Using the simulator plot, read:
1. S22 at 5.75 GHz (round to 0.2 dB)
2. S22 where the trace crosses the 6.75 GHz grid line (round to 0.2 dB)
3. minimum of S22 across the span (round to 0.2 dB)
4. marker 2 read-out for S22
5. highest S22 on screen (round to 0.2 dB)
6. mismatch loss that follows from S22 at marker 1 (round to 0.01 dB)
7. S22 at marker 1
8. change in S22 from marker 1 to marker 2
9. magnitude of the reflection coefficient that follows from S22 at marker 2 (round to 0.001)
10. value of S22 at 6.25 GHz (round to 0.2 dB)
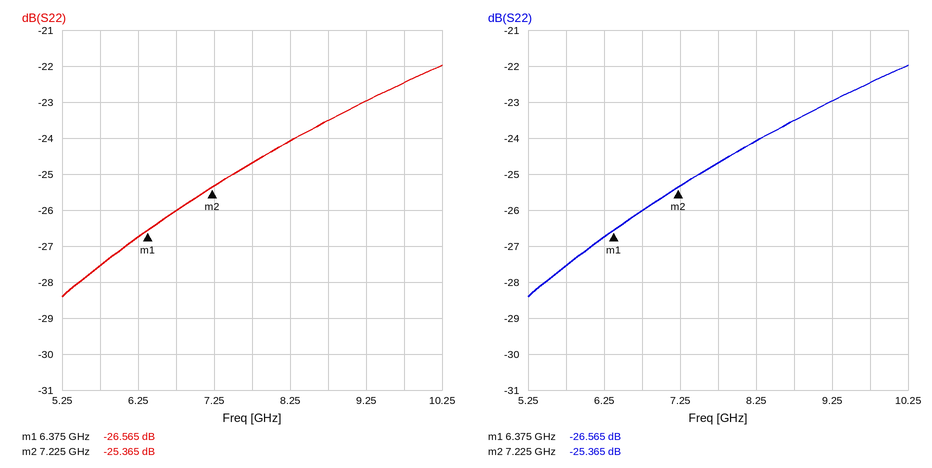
-27.6 dB
-26.0 dB
-28.4 dB
-25.365 dB
-22.0 dB
0.01 dB
-26.565 dB
1.200 dB
0.054
-26.8 dB
